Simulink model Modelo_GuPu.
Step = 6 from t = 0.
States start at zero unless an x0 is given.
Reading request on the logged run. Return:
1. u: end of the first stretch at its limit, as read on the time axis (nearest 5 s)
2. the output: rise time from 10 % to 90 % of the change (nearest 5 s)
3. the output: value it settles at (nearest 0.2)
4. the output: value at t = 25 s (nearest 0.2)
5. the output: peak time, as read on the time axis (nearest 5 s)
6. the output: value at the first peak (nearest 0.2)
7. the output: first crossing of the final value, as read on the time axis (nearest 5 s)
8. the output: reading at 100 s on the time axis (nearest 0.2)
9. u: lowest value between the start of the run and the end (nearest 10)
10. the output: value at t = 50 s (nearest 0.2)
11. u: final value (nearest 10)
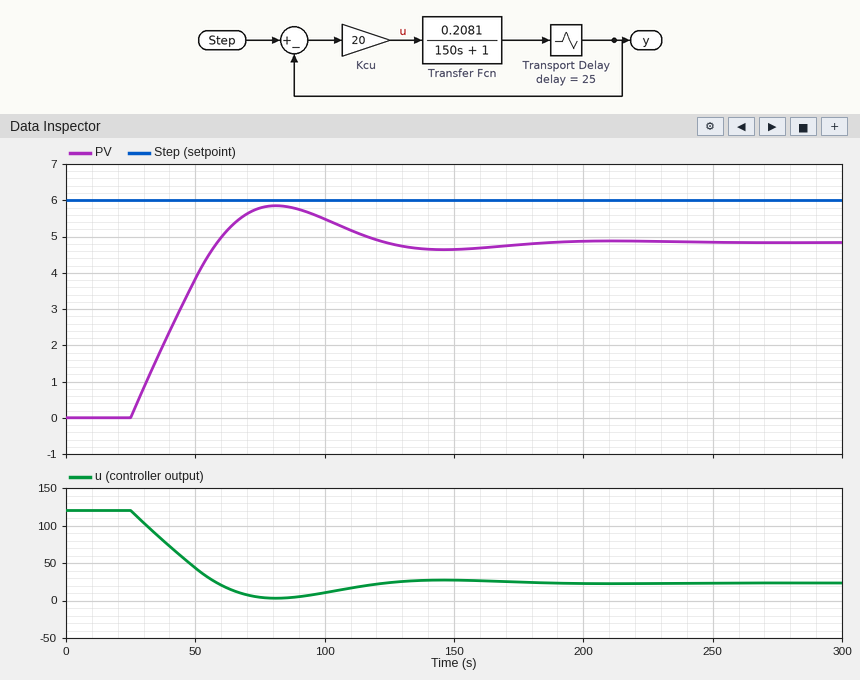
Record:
25 s
25 s
4.8
0.0
80 s
5.8
60 s
5.4
0
3.8
20
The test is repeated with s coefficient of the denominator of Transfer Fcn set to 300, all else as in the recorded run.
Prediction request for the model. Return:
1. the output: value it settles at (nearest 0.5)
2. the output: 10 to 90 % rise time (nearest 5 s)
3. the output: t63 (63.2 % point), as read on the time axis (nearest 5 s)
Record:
5.0
75 s
65 s
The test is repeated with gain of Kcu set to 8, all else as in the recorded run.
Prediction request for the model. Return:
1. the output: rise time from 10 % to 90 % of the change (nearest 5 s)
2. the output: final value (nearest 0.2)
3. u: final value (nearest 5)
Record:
80 s
3.8
20
